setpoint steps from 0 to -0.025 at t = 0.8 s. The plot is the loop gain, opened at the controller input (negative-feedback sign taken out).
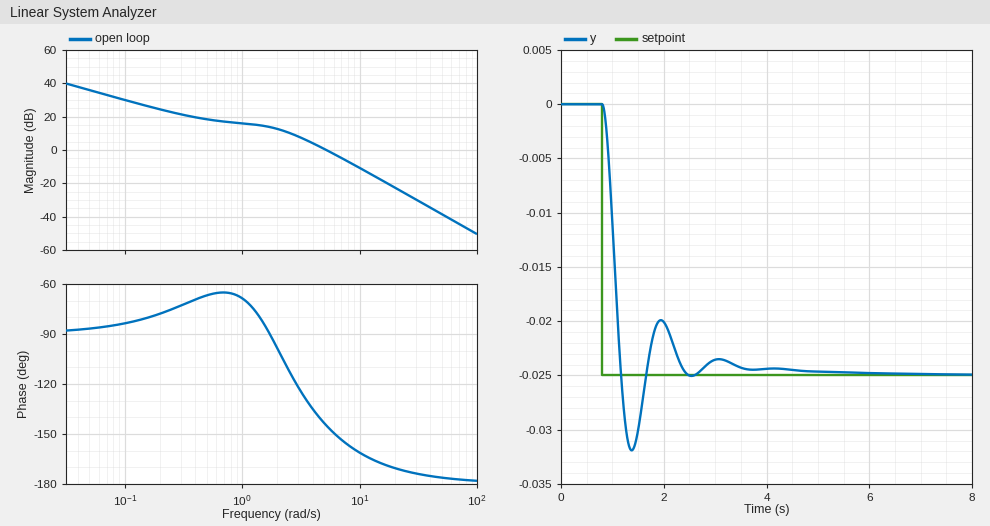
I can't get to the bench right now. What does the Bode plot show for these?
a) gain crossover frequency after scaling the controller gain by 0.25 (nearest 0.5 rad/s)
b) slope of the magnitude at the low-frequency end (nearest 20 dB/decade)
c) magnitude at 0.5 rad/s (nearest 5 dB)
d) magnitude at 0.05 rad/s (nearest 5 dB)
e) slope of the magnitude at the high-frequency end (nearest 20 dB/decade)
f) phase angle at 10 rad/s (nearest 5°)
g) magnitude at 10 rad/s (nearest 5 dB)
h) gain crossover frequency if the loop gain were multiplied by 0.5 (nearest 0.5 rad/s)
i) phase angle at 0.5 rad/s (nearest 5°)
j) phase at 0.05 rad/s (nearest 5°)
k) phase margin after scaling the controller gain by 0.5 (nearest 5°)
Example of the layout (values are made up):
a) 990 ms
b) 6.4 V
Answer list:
a) 2.0 rad/s
b) -20 dB/decade
c) 20 dB
d) 35 dB
e) -40 dB/decade
f) -160°
g) -10 dB
h) 3.5 rad/s
i) -65°
j) -85°
k) 50°
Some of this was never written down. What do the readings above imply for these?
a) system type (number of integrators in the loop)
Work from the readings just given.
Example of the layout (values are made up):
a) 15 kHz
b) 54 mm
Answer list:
a) 1
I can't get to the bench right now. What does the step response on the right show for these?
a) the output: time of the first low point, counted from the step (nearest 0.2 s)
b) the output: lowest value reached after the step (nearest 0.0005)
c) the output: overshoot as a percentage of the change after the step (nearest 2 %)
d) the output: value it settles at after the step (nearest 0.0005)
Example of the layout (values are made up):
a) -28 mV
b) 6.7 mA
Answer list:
a) 0.6 s
b) -0.0320
c) 28 %
d) -0.0250
